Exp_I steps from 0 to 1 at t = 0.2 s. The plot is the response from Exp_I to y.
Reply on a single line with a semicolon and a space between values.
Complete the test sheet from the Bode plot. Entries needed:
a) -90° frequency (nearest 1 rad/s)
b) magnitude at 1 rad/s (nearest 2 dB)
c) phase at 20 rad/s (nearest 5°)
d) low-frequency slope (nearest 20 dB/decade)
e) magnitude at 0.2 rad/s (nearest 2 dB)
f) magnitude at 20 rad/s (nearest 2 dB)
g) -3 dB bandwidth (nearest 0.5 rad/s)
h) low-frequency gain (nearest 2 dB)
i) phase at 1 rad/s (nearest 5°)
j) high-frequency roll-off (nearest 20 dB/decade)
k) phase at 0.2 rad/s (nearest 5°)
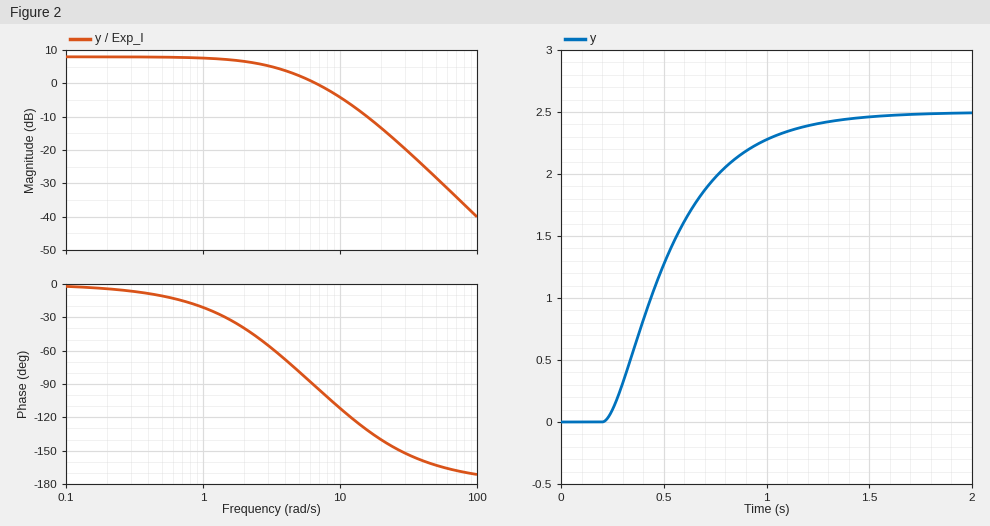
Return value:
6 rad/s; 8 dB; -140°; 0 dB/decade; 8 dB; -14 dB; 3.0 rad/s; 8 dB; -20°; -40 dB/decade; -5°
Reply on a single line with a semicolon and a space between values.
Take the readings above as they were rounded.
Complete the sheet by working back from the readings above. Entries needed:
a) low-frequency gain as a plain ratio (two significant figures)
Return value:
2.5
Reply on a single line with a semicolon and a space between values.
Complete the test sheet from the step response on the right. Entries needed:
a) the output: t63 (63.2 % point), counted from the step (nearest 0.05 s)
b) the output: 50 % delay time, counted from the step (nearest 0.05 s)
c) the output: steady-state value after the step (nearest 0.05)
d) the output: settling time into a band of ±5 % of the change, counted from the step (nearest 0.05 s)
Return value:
0.40 s; 0.30 s; 2.50; 0.95 s
